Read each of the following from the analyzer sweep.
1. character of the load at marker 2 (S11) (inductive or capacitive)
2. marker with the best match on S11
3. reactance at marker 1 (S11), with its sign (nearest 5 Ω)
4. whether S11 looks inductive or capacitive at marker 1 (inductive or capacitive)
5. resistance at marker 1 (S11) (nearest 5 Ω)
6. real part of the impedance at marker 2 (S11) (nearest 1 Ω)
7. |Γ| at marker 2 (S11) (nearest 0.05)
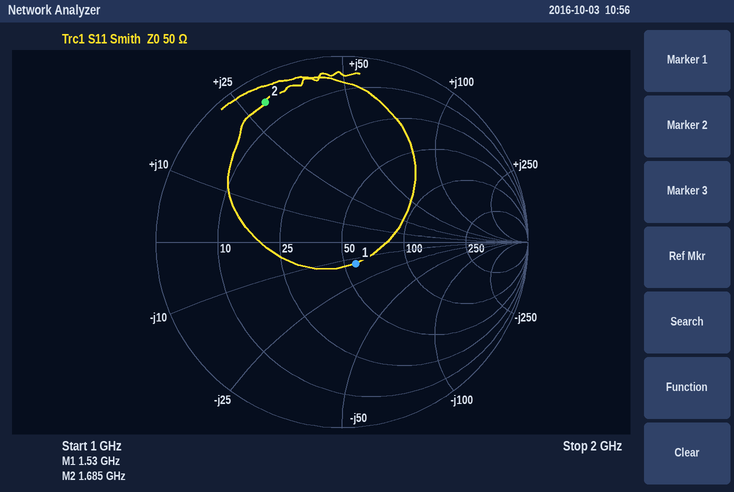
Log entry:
inductive
marker 1
-15 Ω
capacitive
55 Ω
5 Ω
0.85
